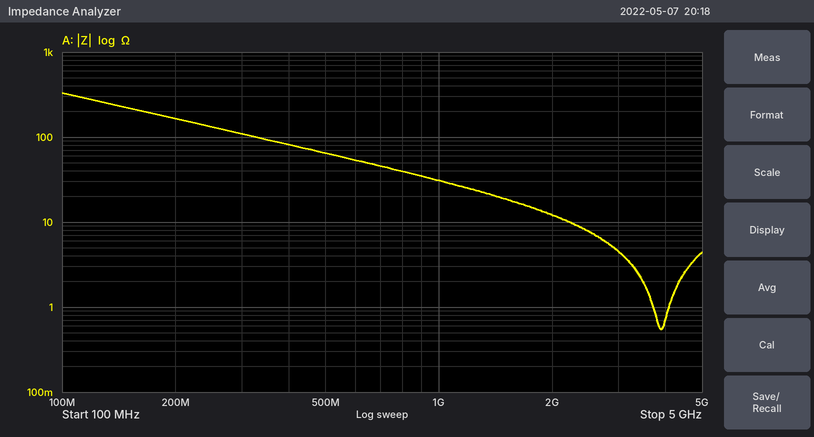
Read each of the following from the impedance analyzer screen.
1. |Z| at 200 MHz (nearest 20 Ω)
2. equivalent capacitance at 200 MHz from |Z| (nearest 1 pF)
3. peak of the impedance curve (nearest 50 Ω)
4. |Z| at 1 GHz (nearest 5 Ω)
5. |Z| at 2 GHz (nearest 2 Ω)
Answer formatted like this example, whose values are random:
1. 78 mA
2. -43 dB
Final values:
1. 160 Ω
2. 5 pF
3. 350 Ω
4. 30 Ω
5. 12 Ω
